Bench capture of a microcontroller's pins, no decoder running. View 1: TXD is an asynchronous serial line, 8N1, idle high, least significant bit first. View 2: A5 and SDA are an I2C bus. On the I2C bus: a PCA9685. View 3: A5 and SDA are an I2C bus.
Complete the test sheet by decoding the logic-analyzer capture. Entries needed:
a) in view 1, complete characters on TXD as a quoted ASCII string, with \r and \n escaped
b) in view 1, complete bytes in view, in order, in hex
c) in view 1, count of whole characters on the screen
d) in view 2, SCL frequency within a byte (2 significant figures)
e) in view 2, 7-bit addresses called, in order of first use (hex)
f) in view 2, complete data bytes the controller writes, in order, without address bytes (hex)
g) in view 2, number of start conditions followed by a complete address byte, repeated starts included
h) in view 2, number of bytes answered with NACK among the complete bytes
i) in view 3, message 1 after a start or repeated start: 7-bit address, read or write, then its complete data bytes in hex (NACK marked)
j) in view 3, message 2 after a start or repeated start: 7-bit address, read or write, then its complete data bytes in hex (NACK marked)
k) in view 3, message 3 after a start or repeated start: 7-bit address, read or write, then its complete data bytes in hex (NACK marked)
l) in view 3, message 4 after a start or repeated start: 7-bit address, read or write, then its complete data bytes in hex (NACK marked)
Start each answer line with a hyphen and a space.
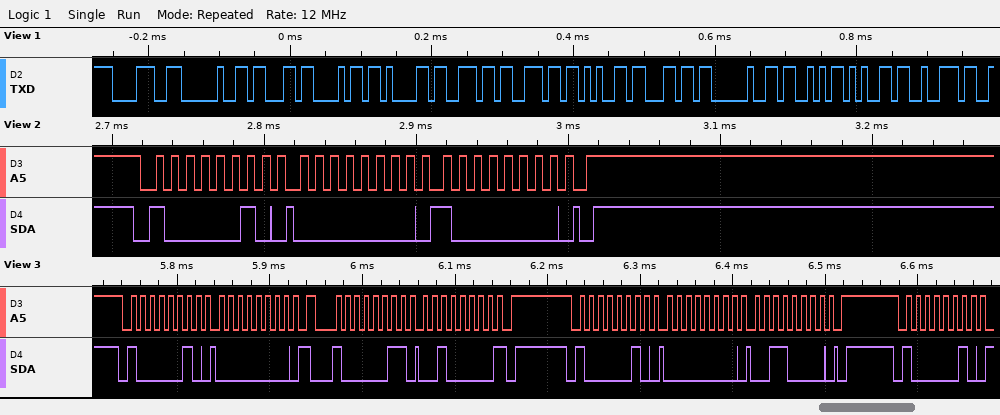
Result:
- "8 channel Ser"
- 0x38 0x20 0x63 0x68 0x61 0x6E 0x6E 0x65 0x6C 0x20 0x53 0x65 0x72
- 13
- 100 kHz
- 0x41
- 00 80
- 1
- 0
- 0x41 write: 00
- 0x41 read: 20 NACK
- 0x41 write: 00 30
- 0x41 write
